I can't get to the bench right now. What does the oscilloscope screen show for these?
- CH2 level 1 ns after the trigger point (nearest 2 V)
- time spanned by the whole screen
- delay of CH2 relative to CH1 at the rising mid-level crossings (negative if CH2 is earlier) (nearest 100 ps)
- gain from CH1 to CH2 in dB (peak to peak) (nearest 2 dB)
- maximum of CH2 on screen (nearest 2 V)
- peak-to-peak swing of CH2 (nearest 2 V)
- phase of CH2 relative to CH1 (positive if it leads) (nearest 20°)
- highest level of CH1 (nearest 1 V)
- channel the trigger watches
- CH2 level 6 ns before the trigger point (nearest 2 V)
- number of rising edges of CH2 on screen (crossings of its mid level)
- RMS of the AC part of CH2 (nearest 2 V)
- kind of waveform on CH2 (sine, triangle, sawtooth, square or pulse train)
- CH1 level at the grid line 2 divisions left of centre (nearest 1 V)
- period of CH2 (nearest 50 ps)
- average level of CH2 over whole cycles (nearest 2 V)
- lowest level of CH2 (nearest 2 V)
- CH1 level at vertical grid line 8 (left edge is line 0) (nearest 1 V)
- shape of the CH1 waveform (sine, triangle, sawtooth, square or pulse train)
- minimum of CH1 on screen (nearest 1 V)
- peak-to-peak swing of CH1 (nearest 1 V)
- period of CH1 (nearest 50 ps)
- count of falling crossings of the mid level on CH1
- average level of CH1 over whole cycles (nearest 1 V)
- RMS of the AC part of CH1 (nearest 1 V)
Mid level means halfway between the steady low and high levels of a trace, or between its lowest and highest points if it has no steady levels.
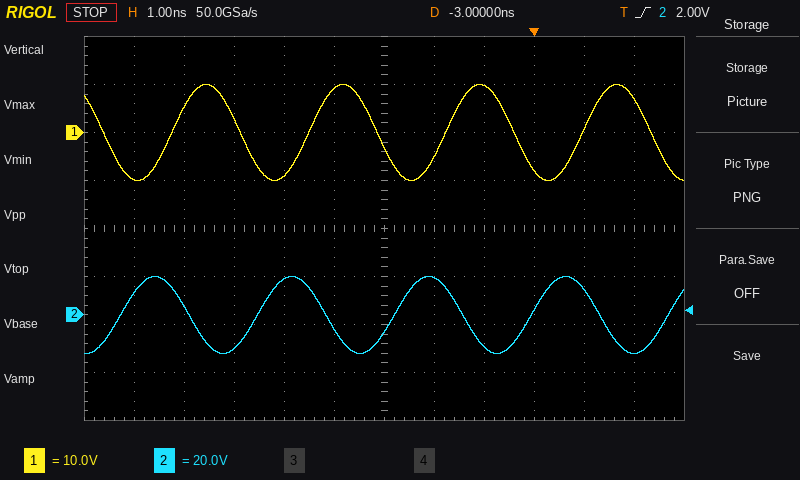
10 V
12 ns
-1.0 ns
4 dB
16 V
32 V
+140°
10 V
CH2
-14 V
5
12 V
sine
-9 V
2.75 ns
0 V
-16 V
10 V
sine
-10 V
20 V
2.75 ns
5
0 V
7 V
